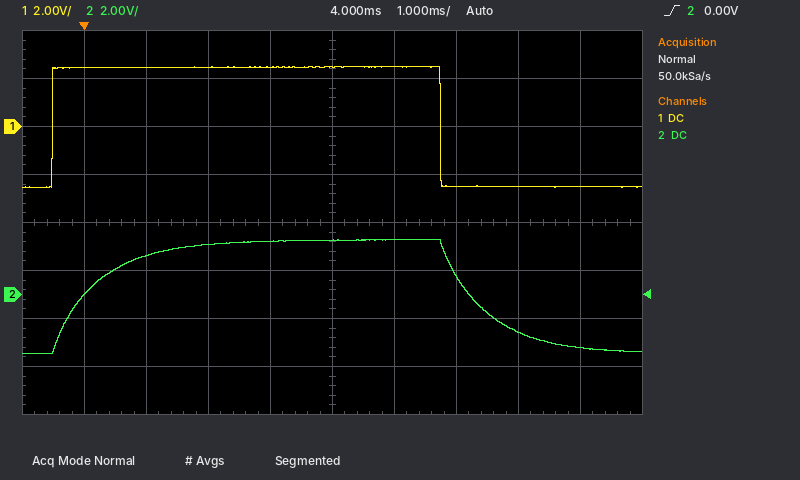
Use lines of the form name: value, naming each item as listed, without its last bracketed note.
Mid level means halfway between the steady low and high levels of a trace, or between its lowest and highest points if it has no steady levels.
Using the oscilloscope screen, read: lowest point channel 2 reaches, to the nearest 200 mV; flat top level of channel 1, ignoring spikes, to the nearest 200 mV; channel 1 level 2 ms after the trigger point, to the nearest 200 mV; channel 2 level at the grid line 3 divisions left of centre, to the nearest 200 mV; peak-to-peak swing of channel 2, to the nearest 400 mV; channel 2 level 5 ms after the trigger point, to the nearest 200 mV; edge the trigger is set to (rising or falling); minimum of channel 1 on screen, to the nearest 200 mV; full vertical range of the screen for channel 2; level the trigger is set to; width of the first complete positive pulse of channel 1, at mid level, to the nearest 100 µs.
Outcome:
lowest point channel 2 reaches, to the nearest 200 mV: -2.4 V
flat top level of channel 1, ignoring spikes, to the nearest 200 mV: 2.4 V
channel 1 level 2 ms after the trigger point, to the nearest 200 mV: 2.4 V
channel 2 level at the grid line 3 divisions left of centre, to the nearest 200 mV: 1.6 V
peak-to-peak swing of channel 2, to the nearest 400 mV: 4.8 V
channel 2 level 5 ms after the trigger point, to the nearest 200 mV: 2.2 V
edge the trigger is set to: rising
minimum of channel 1 on screen, to the nearest 200 mV: -2.6 V
full vertical range of the screen for channel 2: 16 V
level the trigger is set to: 0.00 V
width of the first complete positive pulse of channel 1, at mid level, to the nearest 100 µs: 6.3 ms
